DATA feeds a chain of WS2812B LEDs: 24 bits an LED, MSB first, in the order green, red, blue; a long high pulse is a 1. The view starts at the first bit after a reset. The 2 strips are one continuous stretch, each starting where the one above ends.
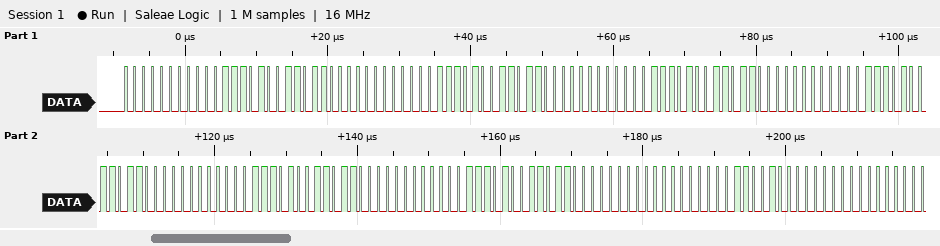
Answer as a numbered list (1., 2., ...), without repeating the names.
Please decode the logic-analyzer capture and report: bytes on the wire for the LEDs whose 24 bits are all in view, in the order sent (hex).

1. 00 1D 36 00 1D 36 00 1D 36 00 1D 36 00 1D 36 00 1D 36 00 00 64
